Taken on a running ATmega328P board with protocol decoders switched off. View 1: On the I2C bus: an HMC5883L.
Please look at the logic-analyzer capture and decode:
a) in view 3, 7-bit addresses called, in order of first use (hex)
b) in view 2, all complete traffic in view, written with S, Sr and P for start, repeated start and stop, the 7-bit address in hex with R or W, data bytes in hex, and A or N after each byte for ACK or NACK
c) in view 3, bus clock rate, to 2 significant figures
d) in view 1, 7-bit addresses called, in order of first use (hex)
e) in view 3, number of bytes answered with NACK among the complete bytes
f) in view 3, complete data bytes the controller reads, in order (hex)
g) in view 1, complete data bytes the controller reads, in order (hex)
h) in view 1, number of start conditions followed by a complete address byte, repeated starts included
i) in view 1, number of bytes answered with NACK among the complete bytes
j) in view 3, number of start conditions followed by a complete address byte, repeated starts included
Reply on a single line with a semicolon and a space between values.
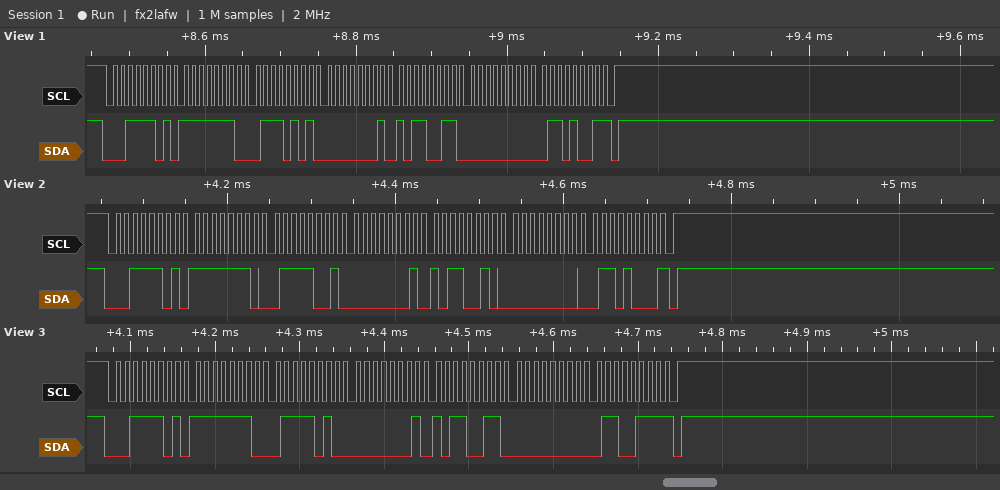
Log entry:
0x1E; S 1ER A FE A 79 A 01 A B2 A 00 A 68 N P; 100 kHz; 0x1E; 1; FE 7A 01 B3 00 67; FE 75 01 B3 00 69; 1; 1; 1
